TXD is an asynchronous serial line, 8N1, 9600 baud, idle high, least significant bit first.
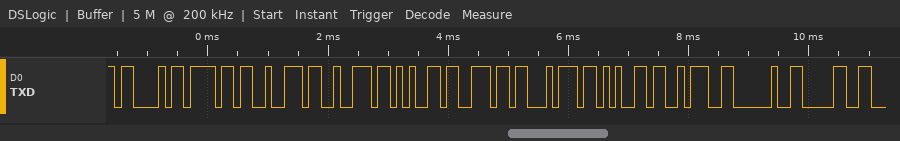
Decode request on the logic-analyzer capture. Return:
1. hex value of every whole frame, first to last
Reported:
0x43 0x6F 0x72 0x72 0x65 0x6E 0x74 0x65 0x3A 0x20 0x30
